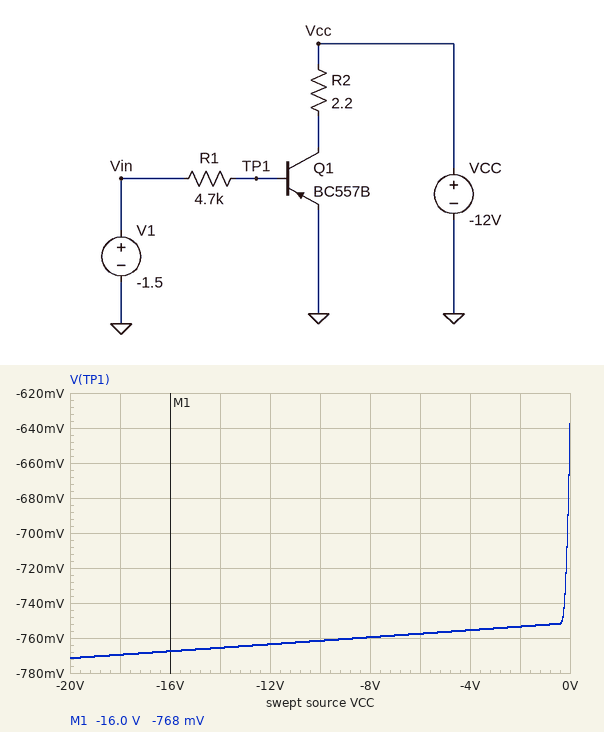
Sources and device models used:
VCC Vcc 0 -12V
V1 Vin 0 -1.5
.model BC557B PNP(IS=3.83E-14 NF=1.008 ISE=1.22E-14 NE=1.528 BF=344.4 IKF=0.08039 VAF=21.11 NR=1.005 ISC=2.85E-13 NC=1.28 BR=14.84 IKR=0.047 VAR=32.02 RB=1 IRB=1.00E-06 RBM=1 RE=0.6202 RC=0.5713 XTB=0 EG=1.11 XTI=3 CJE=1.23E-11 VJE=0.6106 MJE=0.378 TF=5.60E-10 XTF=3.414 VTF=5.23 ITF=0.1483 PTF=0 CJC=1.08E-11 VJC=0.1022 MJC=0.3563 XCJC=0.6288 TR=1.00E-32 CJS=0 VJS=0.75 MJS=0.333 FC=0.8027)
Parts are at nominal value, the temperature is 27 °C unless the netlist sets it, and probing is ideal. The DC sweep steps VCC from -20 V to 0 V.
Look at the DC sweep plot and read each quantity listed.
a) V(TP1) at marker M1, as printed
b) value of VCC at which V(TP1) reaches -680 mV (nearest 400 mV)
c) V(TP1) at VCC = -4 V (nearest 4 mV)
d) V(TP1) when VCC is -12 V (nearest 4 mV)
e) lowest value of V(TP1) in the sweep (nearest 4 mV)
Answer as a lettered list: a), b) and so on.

a) -768 mV
b) 0 V
c) -756 mV
d) -764 mV
e) -772 mV
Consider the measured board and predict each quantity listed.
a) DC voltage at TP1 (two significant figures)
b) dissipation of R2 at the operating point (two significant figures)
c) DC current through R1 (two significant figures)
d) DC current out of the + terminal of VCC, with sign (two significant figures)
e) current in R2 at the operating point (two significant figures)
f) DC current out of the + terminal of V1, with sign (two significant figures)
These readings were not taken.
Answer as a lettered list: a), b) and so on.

a) -760 mV
b) 6.7 mW
c) 160 µA
d) -55 mA
e) 55 mA
f) -160 µA
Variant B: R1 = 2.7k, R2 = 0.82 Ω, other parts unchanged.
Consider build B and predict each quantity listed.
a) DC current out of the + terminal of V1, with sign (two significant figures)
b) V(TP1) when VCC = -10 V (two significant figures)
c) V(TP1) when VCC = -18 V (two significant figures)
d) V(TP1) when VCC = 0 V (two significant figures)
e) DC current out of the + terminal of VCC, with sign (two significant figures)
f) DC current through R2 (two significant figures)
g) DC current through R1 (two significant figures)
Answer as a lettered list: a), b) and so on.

a) -260 µA
b) -790 mV
c) -800 mV
d) -650 mV
e) -81 mA
f) 81 mA
g) 260 µA
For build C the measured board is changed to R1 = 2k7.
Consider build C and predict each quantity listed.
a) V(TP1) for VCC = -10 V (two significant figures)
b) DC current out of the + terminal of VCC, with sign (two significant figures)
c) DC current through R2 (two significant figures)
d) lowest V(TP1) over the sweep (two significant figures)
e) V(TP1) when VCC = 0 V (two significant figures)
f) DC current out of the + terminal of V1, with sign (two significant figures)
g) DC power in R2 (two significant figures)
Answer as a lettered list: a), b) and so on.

a) -790 mV
b) -80 mA
c) 80 mA
d) -800 mV
e) -650 mV
f) -260 µA
g) 14 mW
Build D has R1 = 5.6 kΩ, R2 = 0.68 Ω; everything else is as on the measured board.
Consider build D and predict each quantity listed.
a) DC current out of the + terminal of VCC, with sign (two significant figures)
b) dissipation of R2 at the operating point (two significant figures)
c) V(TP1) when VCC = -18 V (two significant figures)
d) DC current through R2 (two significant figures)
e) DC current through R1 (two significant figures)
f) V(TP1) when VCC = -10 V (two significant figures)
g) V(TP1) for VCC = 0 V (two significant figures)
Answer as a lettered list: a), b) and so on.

a) -49 mA
b) 1.6 mW
c) -760 mV
d) 49 mA
e) 130 µA
f) -750 mV
g) -630 mV
